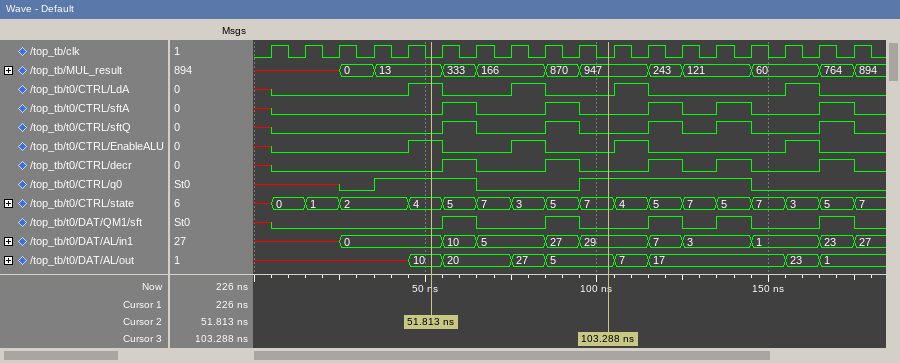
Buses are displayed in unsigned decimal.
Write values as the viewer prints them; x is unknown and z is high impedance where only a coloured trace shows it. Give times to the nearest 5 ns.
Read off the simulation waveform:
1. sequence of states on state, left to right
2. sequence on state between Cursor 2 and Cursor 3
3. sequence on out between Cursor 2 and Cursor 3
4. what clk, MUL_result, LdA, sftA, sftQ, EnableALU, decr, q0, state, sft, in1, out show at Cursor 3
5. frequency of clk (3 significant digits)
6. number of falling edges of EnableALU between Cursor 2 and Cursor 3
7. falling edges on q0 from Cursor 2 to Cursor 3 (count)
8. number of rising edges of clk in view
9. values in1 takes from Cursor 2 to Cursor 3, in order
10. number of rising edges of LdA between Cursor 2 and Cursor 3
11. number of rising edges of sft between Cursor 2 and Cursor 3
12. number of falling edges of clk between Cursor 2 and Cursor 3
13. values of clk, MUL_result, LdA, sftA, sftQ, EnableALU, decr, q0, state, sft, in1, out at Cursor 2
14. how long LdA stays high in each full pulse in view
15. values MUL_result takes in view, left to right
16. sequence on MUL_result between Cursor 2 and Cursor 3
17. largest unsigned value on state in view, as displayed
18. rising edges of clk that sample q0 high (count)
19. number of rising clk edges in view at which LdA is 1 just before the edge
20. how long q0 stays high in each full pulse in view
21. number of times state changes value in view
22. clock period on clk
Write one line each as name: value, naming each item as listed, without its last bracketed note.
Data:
sequence of states on state, left to right: x, 0, 1, 2, 4, 5, 7, 3, 5, 7, 4, 5, 7, 5, 7, 3, 5, 7
sequence on state between Cursor 2 and Cursor 3: 4, 5, 7, 3, 5, 7
sequence on out between Cursor 2 and Cursor 3: 10, 20, 27, 5
what clk, MUL_result, LdA, sftA, sftQ, EnableALU, decr, q0, state, sft, in1, out show at Cursor 3: clk=0, MUL_result=947, LdA=0, sftA=0, sftQ=0, EnableALU=0, decr=0, q0=1, state=7, sft=0, in1=29, out=5
frequency of clk: 100 MHz
number of falling edges of EnableALU between Cursor 2 and Cursor 3: 2
falling edges on q0 from Cursor 2 to Cursor 3: 1
number of rising edges of clk in view: 18
values in1 takes from Cursor 2 to Cursor 3, in order: 0, 10, 5, 27, 29
number of rising edges of LdA between Cursor 2 and Cursor 3: 1
number of rising edges of sft between Cursor 2 and Cursor 3: 2
number of falling edges of clk between Cursor 2 and Cursor 3: 5
values of clk, MUL_result, LdA, sftA, sftQ, EnableALU, decr, q0, state, sft, in1, out at Cursor 2: clk=0, MUL_result=13, LdA=1, sftA=0, sftQ=0, EnableALU=1, decr=0, q0=1, state=4, sft=0, in1=0, out=10
how long LdA stays high in each full pulse in view: 10 ns, 10 ns, 10 ns, 10 ns
values MUL_result takes in view, left to right: x, 0, 13, 333, 166, 870, 947, 243, 121, 60, 764, 894
sequence on MUL_result between Cursor 2 and Cursor 3: 13, 333, 166, 870, 947
largest unsigned value on state in view, as displayed: 7
rising edges of clk that sample q0 high: 8
number of rising clk edges in view at which LdA is 1 just before the edge: 4
how long q0 stays high in each full pulse in view: 30 ns, 50 ns
number of times state changes value in view: 17
clock period on clk: 10 ns
